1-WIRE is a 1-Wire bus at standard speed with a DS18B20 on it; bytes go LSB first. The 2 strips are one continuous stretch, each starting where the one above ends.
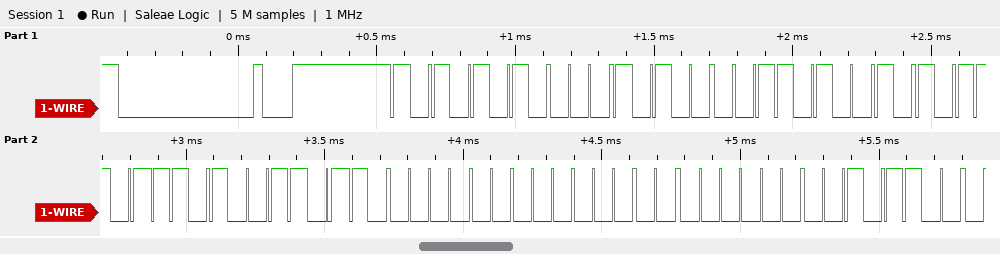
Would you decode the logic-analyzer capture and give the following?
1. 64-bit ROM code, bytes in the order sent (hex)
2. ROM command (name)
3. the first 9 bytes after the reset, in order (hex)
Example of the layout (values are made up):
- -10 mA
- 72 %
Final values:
- 28 2C B5 CB 06 00 00 34
- Match ROM
- 55 28 2C B5 CB 06 00 00 34
